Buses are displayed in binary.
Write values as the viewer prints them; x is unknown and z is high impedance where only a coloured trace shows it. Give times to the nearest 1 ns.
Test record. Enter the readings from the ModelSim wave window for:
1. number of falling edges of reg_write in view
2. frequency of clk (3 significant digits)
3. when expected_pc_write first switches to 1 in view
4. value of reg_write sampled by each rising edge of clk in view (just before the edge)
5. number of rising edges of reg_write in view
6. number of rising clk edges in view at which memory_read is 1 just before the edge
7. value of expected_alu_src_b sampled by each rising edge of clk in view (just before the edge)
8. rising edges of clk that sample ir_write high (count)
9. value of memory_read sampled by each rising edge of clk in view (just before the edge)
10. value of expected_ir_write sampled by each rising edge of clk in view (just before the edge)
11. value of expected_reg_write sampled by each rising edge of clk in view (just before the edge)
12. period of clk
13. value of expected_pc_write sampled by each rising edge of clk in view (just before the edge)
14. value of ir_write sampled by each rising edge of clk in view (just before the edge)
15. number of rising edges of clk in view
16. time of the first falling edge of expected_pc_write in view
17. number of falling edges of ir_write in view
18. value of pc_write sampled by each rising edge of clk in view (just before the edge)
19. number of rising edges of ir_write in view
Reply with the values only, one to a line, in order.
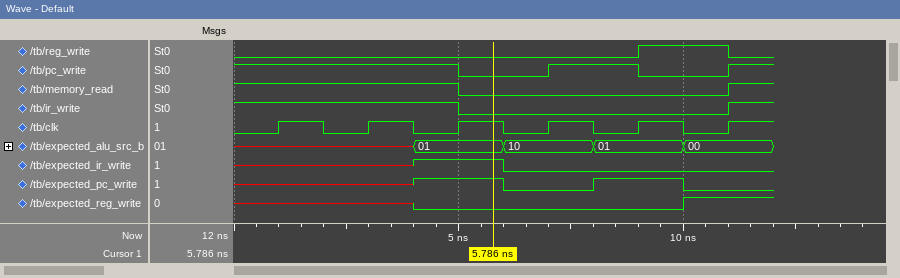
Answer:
1
500 MHz
4 ns
0 0 0 0 0 1
1
3
x, x, 01, 10, 01, 00
3
1 1 1 0 0 0
x x 1 0 0 0
x x 0 0 0 1
2 ns
x x 1 0 1 0
1 1 1 0 0 0
6
6 ns
1
1 1 1 0 1 0
1
